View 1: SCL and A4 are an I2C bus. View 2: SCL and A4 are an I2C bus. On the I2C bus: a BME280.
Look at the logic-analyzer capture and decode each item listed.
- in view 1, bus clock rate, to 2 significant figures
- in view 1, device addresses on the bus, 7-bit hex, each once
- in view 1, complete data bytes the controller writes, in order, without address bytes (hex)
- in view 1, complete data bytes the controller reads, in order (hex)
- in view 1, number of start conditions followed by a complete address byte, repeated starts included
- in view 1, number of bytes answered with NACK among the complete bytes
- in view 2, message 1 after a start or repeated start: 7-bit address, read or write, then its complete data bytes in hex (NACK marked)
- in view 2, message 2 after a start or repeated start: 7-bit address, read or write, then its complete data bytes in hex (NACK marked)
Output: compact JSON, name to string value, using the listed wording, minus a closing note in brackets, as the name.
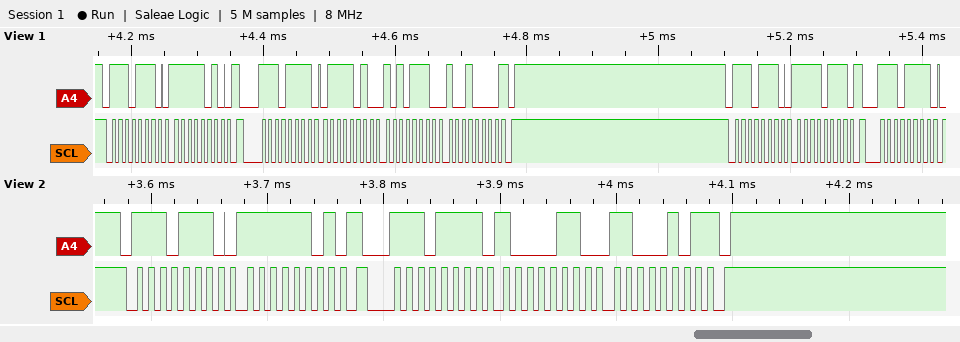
{"in view 1, bus clock rate, to 2 significant figures": "100 kHz", "in view 1, device addresses on the bus, 7-bit hex, each once": "0x77", "in view 1, complete data bytes the controller writes, in order, without address bytes": "FA F7", "in view 1, complete data bytes the controller reads, in order": "7A AE 90", "in view 1, number of start conditions followed by a complete address byte, repeated starts included": "4", "in view 1, number of bytes answered with NACK among the complete bytes": "1", "in view 2, message 1 after a start or repeated start: 7-bit address, read or write, then its complete data bytes in hex": "0x77 write: FD", "in view 2, message 2 after a start or repeated start: 7-bit address, read or write, then its complete data bytes in hex": "0x77 read: 86 C5 NACK"}
